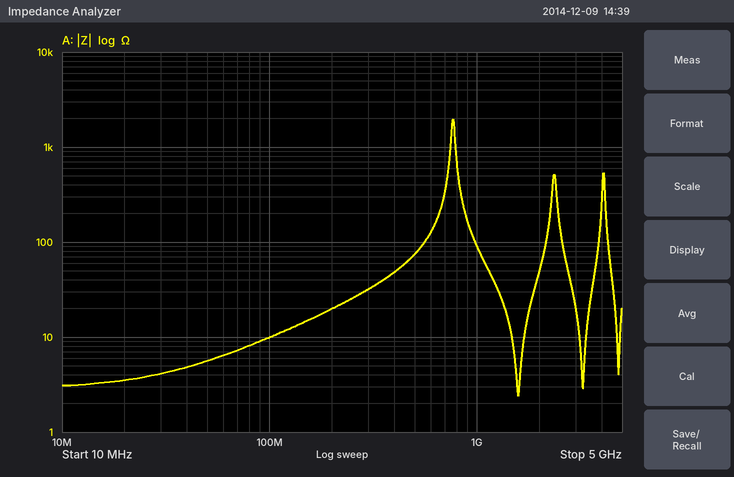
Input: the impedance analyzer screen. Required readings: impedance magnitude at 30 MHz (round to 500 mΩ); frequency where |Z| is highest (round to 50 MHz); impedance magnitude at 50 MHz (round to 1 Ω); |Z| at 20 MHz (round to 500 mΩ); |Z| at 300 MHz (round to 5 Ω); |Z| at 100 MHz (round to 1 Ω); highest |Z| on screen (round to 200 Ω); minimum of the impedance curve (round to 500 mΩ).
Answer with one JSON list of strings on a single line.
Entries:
["4.0 Ω", "750 MHz", "6 Ω", "3.5 Ω", "30 Ω", "10 Ω", "2.0 kΩ", "2.5 Ω"]
